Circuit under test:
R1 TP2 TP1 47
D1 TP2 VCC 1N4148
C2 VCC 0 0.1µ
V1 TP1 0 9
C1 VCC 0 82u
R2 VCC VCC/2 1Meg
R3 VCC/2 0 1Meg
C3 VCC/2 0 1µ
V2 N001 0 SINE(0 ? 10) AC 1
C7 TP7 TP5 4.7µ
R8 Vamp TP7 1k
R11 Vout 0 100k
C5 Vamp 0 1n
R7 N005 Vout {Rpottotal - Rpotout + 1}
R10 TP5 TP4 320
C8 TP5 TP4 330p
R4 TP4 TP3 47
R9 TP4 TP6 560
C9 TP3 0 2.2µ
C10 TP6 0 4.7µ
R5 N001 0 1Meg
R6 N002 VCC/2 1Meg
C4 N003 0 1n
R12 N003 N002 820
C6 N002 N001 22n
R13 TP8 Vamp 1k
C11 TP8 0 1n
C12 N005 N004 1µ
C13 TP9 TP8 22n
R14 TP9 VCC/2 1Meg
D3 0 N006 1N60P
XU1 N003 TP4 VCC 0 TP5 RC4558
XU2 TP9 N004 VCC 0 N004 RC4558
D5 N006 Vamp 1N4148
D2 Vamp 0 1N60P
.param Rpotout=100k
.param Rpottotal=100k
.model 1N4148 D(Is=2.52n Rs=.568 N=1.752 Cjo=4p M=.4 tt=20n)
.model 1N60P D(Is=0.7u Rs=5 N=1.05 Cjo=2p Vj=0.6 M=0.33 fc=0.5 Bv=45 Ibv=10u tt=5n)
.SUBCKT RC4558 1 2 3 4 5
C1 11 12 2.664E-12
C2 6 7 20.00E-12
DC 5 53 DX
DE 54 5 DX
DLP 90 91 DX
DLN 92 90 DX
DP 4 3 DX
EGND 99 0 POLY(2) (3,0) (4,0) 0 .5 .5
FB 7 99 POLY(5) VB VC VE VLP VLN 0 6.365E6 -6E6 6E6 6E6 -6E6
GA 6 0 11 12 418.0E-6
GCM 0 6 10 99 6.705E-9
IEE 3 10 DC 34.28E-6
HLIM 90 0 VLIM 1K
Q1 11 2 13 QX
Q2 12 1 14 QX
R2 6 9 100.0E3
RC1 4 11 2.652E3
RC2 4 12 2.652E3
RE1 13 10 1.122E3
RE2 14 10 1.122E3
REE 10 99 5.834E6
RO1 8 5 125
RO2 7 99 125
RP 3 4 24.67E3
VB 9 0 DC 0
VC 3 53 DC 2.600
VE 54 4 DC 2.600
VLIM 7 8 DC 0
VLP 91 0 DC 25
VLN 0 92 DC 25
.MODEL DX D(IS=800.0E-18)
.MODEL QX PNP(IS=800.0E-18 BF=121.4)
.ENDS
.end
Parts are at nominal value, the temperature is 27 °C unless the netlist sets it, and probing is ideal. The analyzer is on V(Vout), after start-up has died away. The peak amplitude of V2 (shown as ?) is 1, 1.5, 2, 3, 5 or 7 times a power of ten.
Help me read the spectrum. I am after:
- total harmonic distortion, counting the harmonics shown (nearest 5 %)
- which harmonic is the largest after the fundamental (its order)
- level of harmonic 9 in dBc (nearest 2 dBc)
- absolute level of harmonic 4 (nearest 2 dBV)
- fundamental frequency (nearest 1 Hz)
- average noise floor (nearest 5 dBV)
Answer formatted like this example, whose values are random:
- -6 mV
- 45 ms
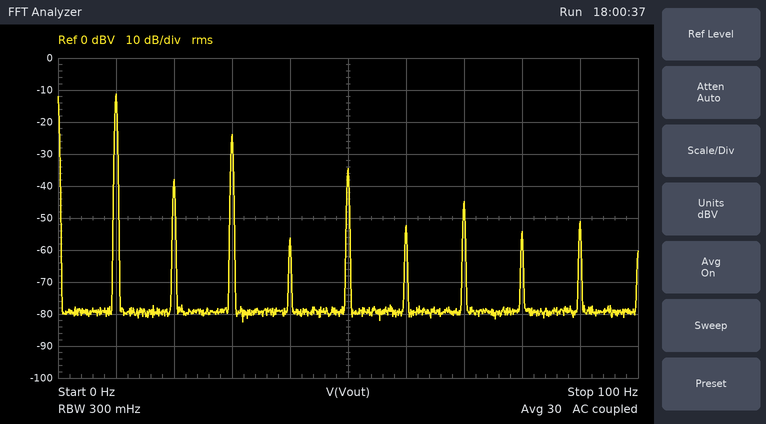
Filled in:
- 25 %
- 3
- -40 dBc
- -56 dBV
- 10 Hz
- -80 dBV
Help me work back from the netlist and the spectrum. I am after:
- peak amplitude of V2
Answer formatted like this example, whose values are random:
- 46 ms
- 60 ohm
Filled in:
- 1.5 V
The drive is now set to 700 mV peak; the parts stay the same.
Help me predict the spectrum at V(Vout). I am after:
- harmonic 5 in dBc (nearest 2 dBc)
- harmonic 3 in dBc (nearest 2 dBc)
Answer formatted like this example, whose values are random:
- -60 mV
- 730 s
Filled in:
- -34 dBc
- -18 dBc
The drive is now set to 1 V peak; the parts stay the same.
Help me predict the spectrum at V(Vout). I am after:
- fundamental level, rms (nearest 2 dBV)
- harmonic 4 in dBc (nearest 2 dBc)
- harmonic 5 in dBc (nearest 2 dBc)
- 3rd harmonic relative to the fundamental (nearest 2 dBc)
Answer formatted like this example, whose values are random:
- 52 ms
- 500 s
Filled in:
- -12 dBV
- -40 dBc
- -28 dBc
- -14 dBc
